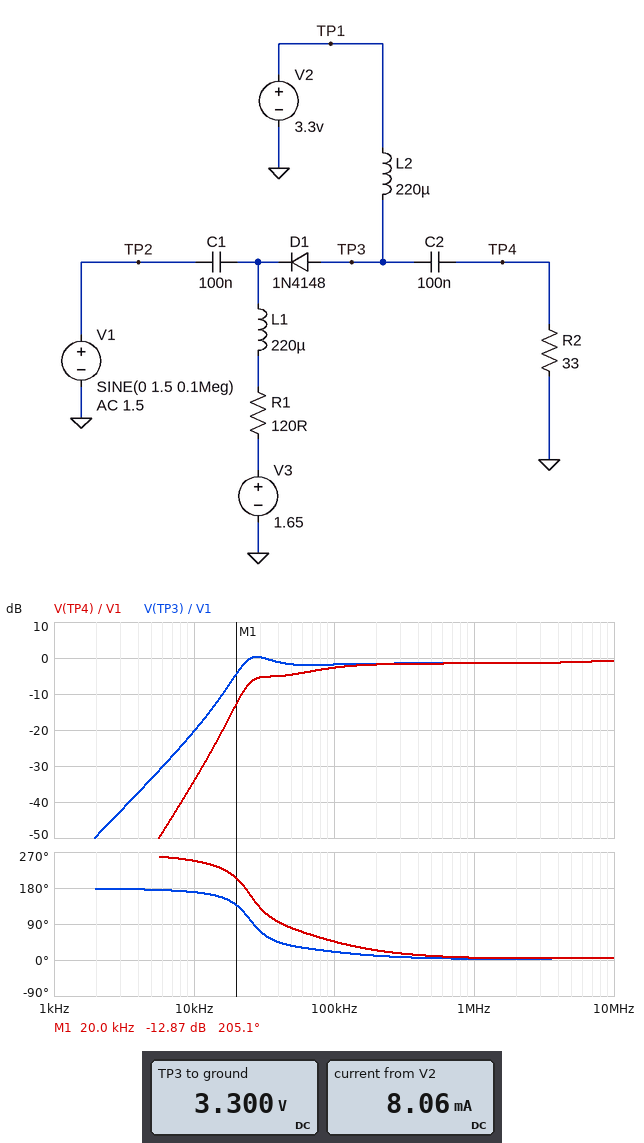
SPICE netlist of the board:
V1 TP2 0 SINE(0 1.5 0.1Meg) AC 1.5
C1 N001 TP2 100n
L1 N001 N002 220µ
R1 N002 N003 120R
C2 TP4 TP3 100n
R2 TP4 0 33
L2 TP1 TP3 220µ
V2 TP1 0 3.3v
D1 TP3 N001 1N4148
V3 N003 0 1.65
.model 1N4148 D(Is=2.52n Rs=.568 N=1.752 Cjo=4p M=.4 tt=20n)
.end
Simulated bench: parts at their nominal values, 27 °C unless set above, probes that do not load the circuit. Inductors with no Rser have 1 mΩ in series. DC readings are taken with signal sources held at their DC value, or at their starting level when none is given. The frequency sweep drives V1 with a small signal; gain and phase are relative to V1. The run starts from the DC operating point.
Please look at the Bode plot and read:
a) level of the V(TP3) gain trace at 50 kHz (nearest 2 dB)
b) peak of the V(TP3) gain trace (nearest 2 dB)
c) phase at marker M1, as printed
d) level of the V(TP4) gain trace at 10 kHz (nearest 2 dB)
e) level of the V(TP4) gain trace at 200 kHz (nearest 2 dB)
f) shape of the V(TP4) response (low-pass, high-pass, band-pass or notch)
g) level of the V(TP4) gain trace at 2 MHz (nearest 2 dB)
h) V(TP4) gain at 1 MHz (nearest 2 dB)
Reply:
-2 dB
0 dB
205.1 deg
-34 dB
-2 dB
high-pass
-2 dB
-2 dB
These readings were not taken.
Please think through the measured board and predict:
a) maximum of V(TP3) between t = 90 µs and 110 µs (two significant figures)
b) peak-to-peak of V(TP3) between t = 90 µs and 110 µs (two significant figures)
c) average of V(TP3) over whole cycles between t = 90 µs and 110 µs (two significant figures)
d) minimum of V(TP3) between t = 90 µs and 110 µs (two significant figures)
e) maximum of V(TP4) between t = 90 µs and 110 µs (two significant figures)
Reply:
3.8 V
1.5 V
3.3 V
2.3 V
550 mV
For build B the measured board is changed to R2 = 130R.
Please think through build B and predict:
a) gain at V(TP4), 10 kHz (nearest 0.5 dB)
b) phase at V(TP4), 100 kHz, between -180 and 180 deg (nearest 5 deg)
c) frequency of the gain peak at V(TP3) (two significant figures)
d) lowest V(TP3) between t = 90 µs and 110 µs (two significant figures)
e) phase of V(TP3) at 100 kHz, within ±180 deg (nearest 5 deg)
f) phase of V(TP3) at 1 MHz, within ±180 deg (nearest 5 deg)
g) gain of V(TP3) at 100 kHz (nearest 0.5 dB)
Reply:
-24.5 dB
20 deg
42 kHz
1.9 V
15 deg
0 deg
1.0 dB
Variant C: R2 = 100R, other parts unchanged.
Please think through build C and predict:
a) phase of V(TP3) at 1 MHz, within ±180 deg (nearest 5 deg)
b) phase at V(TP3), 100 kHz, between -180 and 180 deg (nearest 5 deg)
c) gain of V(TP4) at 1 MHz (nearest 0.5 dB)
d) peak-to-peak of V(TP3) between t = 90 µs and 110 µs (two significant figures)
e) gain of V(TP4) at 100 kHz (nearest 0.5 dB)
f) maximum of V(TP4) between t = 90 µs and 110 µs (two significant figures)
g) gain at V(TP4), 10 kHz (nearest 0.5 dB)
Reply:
0 deg
15 deg
-0.5 dB
2.7 V
0.5 dB
1.4 V
-26.0 dB
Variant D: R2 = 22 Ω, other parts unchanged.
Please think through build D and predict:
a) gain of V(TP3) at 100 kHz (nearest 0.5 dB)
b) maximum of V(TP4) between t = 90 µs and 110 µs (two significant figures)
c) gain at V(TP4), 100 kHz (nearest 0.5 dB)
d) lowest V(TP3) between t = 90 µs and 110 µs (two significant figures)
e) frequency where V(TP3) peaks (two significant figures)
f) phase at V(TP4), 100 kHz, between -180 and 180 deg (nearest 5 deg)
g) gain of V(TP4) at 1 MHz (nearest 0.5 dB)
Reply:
-3.0 dB
360 mV
-5.0 dB
2.5 V
27 kHz
55 deg
-2.0 dB
